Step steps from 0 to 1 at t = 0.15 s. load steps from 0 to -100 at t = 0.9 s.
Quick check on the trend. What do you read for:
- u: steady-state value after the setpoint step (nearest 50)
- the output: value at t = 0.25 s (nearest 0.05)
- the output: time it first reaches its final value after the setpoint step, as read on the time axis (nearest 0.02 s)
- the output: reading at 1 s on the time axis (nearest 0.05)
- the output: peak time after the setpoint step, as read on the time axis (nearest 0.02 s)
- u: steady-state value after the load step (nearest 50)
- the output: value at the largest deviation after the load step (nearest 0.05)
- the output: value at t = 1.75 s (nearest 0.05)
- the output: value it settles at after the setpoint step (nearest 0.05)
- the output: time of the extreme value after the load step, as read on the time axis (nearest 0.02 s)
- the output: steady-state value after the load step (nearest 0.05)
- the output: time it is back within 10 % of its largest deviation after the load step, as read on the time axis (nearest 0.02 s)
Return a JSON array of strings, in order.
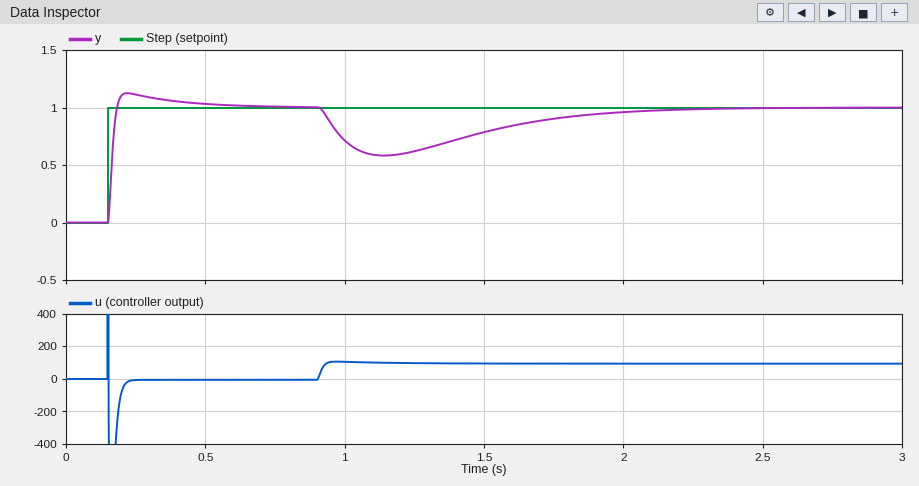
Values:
["0", "1.10", "0.18 s", "0.70", "0.22 s", "100", "0.60", "0.90", "1.00", "1.14 s", "1.00", "1.98 s"]
